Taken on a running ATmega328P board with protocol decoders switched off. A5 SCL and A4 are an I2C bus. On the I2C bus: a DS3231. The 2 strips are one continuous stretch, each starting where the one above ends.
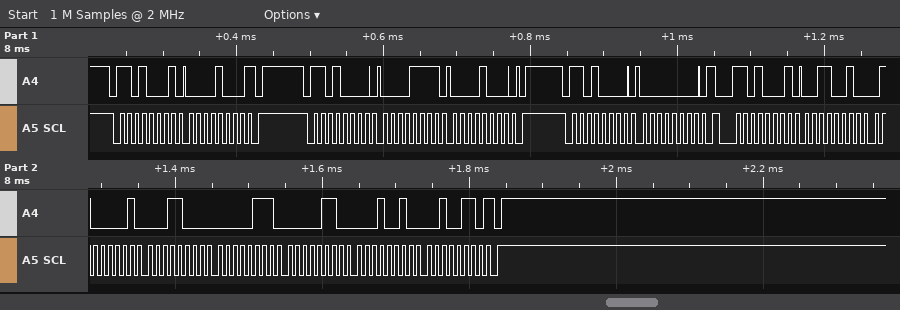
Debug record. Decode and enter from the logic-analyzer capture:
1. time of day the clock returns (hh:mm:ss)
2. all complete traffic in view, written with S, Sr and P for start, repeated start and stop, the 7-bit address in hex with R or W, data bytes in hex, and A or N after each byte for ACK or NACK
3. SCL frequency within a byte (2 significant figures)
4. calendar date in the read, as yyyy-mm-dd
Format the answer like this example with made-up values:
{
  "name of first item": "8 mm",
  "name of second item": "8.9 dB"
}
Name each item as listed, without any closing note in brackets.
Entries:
{
  "time of day the clock returns": "18:41:32",
  "all complete traffic in view, written with S, Sr and P for start, repeated start and stop, the 7-bit address in hex with R or W, data bytes in hex, and A or N after each byte for ACK or NACK": "S 68R A 08 N P S 68W A 0F A 08 A P S 68W A 00 A Sr 68R A 32 A 41 A 18 A 07 A 06 A 12 A 26 N P",
  "SCL frequency within a byte": "100 kHz",
  "calendar date in the read, as yyyy-mm-dd": "2026-12-06"
}
